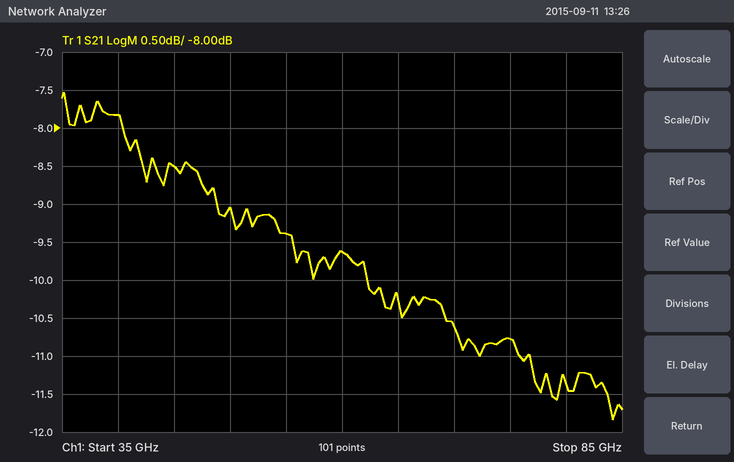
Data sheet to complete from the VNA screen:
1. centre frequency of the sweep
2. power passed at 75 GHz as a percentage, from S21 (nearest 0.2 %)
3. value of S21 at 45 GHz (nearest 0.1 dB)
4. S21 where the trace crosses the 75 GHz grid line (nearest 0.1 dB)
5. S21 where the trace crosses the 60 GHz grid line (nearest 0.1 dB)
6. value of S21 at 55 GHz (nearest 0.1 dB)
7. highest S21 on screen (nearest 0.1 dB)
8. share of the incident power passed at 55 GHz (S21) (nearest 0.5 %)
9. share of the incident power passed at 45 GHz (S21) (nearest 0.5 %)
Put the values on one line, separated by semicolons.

60 GHz; 8.4 %; -8.5 dB; -10.8 dB; -9.6 dB; -9.4 dB; -7.5 dB; 11.5 %; 14.0 %
